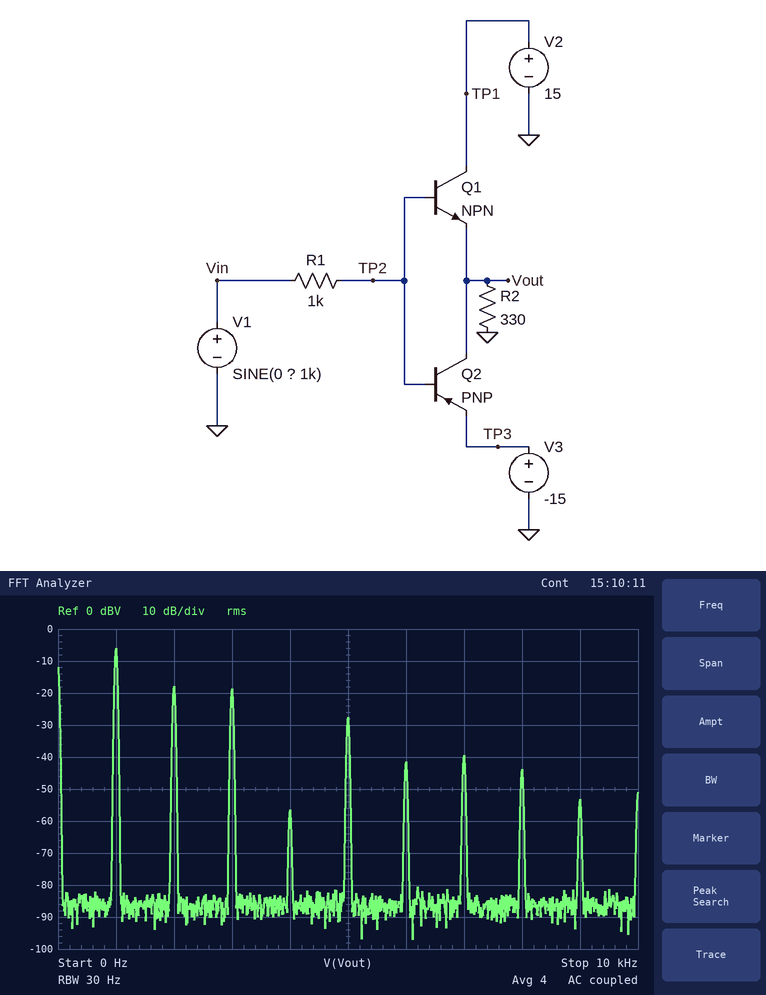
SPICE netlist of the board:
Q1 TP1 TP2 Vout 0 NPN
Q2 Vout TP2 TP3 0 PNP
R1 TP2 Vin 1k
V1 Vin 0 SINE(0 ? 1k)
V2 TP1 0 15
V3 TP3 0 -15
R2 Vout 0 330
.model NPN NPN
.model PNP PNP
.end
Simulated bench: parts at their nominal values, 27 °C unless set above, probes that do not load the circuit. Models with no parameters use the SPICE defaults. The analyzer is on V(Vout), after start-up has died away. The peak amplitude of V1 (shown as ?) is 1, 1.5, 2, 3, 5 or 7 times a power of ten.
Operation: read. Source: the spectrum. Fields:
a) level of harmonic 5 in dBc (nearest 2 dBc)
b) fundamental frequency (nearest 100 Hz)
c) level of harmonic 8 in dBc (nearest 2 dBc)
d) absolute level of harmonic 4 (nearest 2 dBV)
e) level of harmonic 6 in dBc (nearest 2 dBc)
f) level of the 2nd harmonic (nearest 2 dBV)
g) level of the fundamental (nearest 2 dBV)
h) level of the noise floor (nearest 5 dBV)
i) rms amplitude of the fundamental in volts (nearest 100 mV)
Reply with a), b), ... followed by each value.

a) -22 dBc
b) 1.0 kHz
c) -38 dBc
d) -56 dBV
e) -36 dBc
f) -18 dBV
g) -6 dBV
h) -85 dBV
i) 500 mV
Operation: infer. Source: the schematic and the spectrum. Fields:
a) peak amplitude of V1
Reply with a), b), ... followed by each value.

a) 2 V
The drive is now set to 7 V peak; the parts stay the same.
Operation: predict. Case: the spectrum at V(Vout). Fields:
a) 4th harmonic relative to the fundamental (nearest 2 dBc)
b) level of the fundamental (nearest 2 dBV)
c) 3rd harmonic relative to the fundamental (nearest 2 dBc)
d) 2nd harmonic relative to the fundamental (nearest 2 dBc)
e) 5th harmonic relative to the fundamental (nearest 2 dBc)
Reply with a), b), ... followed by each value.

a) -28 dBc
b) 10 dBV
c) -26 dBc
d) -14 dBc
e) -30 dBc
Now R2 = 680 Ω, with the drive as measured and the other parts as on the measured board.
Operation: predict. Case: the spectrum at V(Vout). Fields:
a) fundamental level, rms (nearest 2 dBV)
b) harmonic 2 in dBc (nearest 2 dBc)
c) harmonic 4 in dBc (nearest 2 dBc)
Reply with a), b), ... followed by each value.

a) -4 dBV
b) -16 dBc
c) -54 dBc
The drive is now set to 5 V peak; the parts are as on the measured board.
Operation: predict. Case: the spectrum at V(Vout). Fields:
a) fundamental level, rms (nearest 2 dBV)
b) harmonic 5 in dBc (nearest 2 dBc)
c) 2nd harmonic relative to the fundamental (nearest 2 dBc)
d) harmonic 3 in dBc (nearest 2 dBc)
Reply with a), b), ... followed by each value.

a) 6 dBV
b) -28 dBc
c) -14 dBc
d) -22 dBc
